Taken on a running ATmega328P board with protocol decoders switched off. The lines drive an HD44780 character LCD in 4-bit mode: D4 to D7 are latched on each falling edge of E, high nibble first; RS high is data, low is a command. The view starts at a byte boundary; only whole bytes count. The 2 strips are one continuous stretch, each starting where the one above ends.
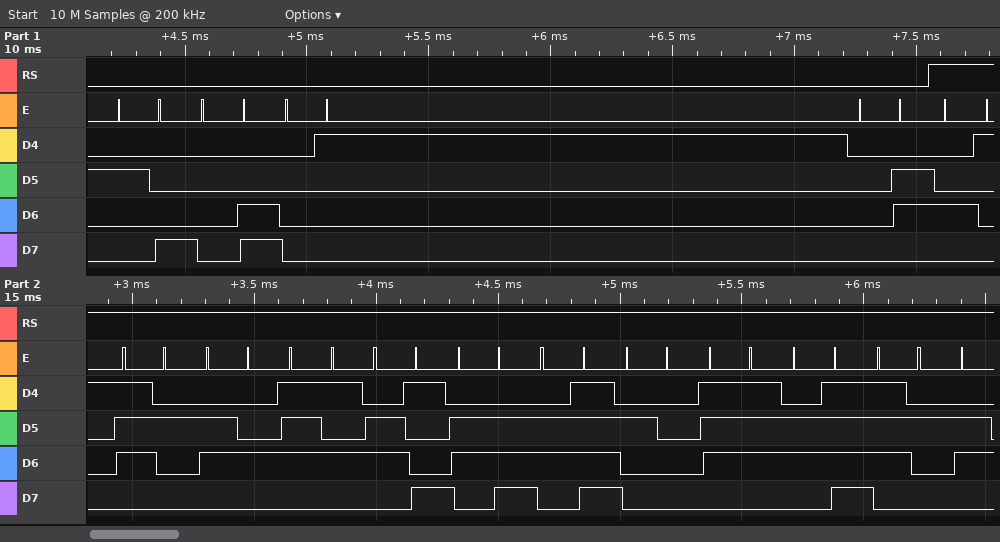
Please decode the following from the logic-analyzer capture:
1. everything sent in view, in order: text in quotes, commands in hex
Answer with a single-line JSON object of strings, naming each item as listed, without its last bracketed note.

{"everything sent in view, in order: text in quotes, commands in hex": "0x28 0x0C 0x01 0x06 \"Arduino wor\""}
